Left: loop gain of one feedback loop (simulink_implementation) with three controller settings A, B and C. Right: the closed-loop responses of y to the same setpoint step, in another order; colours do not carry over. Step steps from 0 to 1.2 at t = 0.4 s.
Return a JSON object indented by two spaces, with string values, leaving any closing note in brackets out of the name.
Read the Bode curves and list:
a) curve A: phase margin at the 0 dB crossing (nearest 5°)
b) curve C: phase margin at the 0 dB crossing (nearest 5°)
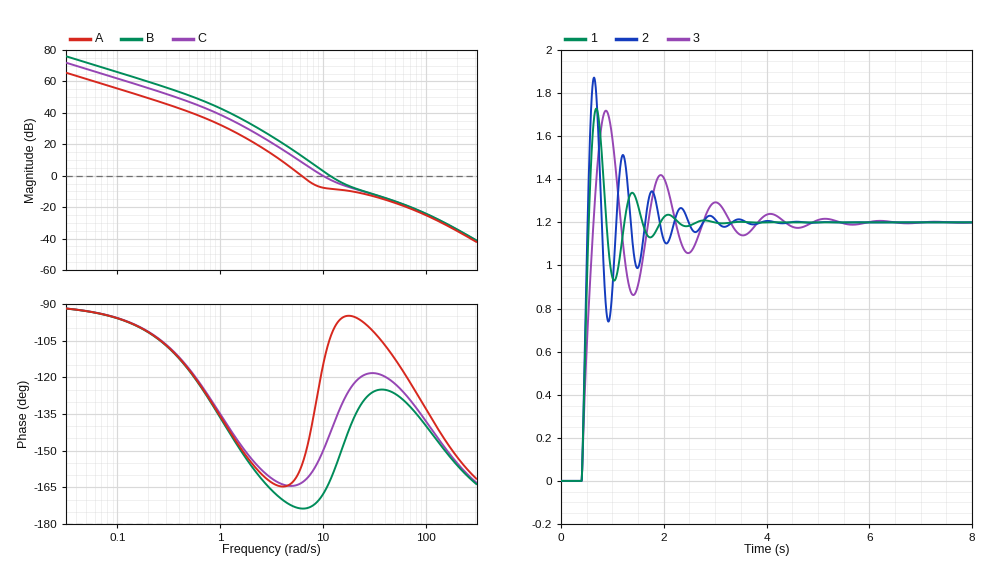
{
  "curve A: phase margin at the 0 dB crossing": "25°",
  "curve C: phase margin at the 0 dB crossing": "30°"
}
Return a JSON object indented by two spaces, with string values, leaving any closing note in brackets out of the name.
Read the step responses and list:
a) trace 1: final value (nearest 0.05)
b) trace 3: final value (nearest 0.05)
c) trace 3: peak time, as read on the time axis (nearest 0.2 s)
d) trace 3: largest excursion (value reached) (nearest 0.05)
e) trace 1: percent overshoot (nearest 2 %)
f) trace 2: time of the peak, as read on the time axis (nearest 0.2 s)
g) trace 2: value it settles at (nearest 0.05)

{
  "trace 1: final value": "1.20",
  "trace 3: final value": "1.20",
  "trace 3: peak time, as read on the time axis": "0.8 s",
  "trace 3: largest excursion (value reached)": "1.70",
  "trace 1: percent overshoot": "44 %",
  "trace 2: time of the peak, as read on the time axis": "0.6 s",
  "trace 2: value it settles at": "1.20"
}
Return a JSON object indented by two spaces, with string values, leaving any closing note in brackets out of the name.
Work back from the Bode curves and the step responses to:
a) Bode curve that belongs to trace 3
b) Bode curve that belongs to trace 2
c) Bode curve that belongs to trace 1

{
  "Bode curve that belongs to trace 3": "A",
  "Bode curve that belongs to trace 2": "B",
  "Bode curve that belongs to trace 1": "C"
}
